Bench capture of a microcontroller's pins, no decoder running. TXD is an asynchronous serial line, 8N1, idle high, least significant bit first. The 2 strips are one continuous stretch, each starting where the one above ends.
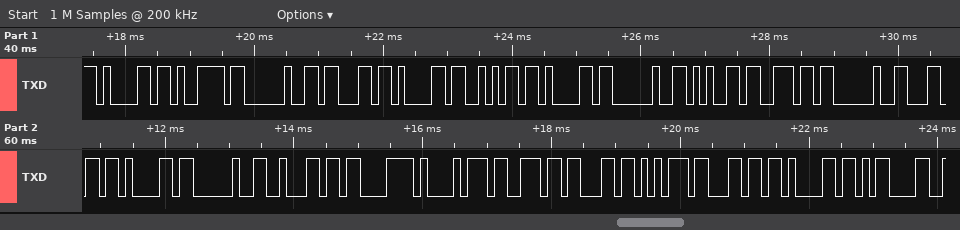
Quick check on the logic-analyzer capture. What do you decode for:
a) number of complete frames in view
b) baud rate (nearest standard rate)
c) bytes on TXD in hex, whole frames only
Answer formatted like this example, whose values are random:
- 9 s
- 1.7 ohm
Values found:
- 23
- 9600 baud
- 0x61 0x79 0x20 0x63 0x61 0x6A 0x61 0x20 0x65 0x6E 0x20 0x6C 0x61 0x20 0x62 0xC3 0xA1 0x73 0x63 0x75 0x6C 0x61 0x0D
